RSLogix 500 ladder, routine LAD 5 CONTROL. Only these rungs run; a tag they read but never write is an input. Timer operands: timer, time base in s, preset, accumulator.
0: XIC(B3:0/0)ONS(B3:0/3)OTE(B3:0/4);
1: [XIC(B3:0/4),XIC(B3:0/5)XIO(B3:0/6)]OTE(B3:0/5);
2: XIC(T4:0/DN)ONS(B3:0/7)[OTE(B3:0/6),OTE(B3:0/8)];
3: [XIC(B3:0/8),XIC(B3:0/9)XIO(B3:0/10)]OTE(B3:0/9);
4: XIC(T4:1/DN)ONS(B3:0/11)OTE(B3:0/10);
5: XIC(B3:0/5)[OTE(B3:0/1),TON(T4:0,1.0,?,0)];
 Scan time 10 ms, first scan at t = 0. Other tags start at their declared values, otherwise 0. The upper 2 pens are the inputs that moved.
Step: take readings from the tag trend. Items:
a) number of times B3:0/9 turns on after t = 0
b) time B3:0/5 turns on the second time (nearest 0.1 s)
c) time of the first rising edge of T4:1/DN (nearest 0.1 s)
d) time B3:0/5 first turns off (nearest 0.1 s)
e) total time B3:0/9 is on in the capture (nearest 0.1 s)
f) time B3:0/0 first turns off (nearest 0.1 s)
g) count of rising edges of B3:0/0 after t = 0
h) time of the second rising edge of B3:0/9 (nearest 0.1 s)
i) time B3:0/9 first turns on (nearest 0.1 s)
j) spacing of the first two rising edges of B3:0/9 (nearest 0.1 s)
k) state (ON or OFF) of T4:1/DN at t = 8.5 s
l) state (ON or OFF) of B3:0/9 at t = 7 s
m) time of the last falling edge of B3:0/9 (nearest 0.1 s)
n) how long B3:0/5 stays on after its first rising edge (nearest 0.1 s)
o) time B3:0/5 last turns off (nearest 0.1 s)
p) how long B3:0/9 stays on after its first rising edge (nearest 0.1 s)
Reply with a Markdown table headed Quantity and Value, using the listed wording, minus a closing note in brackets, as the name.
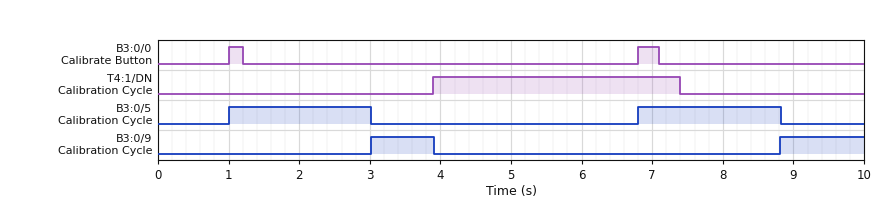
| Quantity | Value |
|---|---|
| number of times B3:0/9 turns on after t = 0 | 2 |
| time B3:0/5 turns on the second time | 6.8 s |
| time of the first rising edge of T4:1/DN | 3.9 s |
| time B3:0/5 first turns off | 3.0 s |
| total time B3:0/9 is on in the capture | 2.1 s |
| time B3:0/0 first turns off | 1.2 s |
| count of rising edges of B3:0/0 after t = 0 | 2 |
| time of the second rising edge of B3:0/9 | 8.8 s |
| time B3:0/9 first turns on | 3.0 s |
| spacing of the first two rising edges of B3:0/9 | 5.8 s |
| state (ON or OFF) of T4:1/DN at t = 8.5 s | OFF |
| state (ON or OFF) of B3:0/9 at t = 7 s | OFF |
| time of the last falling edge of B3:0/9 | 3.9 s |
| how long B3:0/5 stays on after its first rising edge | 2.0 s |
| time B3:0/5 last turns off | 8.8 s |
| how long B3:0/9 stays on after its first rising edge | 0.9 s |
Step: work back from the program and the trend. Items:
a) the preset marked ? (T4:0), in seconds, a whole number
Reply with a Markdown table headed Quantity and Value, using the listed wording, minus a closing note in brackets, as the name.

| Quantity | Value |
|---|---|
| the preset marked ? (T4:0), in seconds, a whole number | 2 s |
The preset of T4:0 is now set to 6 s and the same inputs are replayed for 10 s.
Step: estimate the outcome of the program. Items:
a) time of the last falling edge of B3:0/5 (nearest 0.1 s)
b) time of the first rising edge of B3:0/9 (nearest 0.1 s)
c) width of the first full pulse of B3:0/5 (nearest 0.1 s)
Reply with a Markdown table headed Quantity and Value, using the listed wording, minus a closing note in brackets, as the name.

| Quantity | Value |
|---|---|
| time of the last falling edge of B3:0/5 | 7.0 s |
| time of the first rising edge of B3:0/9 | 7.0 s |
| width of the first full pulse of B3:0/5 | 6.0 s |
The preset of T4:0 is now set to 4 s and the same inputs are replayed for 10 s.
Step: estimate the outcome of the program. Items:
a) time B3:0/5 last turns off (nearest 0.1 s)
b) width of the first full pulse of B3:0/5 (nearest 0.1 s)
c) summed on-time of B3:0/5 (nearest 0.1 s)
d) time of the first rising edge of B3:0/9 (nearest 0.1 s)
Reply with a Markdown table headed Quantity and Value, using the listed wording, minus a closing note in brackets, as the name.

| Quantity | Value |
|---|---|
| time B3:0/5 last turns off | 5.0 s |
| width of the first full pulse of B3:0/5 | 4.0 s |
| summed on-time of B3:0/5 | 7.2 s |
| time of the first rising edge of B3:0/9 | 5.0 s |
